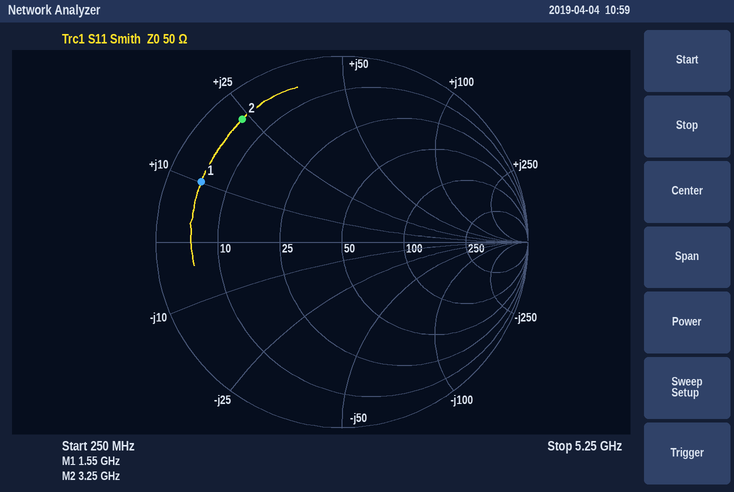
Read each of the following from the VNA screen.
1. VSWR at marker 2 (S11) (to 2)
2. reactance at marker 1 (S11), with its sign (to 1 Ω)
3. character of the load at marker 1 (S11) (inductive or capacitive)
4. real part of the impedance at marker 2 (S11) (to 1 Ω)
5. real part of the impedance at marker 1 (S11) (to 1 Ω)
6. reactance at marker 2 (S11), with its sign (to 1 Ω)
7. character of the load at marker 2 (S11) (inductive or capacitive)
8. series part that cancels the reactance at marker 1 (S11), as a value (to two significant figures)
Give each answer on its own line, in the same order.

12
+10 Ω
inductive
5 Ω
5 Ω
+24 Ω
inductive
10 pF
